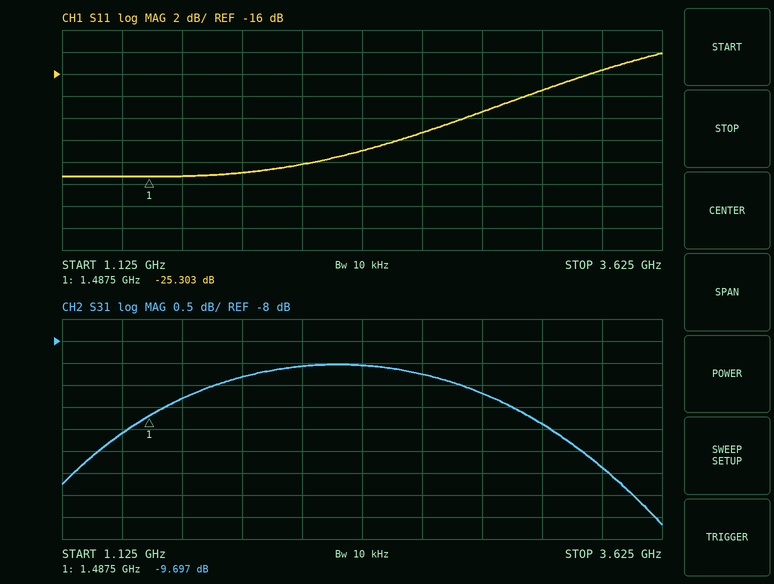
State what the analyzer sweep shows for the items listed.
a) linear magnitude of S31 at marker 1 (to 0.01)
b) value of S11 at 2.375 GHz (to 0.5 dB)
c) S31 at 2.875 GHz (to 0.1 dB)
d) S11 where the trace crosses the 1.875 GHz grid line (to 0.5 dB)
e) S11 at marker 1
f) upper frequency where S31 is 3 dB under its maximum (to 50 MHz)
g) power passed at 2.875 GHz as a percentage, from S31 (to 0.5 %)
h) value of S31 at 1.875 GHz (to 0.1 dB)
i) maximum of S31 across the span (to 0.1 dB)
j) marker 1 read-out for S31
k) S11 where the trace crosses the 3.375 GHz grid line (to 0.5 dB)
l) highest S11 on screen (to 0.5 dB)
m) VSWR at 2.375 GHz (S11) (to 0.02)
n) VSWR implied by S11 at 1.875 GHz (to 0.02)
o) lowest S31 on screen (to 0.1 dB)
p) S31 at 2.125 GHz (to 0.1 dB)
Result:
0.33
-23.0 dB
-9.2 dB
-25.0 dB
-25.303 dB
3.50 GHz
12.0 %
-8.8 dB
-8.5 dB
-9.697 dB
-15.5 dB
-14.0 dB
1.16
1.12
-12.2 dB
-8.6 dB
